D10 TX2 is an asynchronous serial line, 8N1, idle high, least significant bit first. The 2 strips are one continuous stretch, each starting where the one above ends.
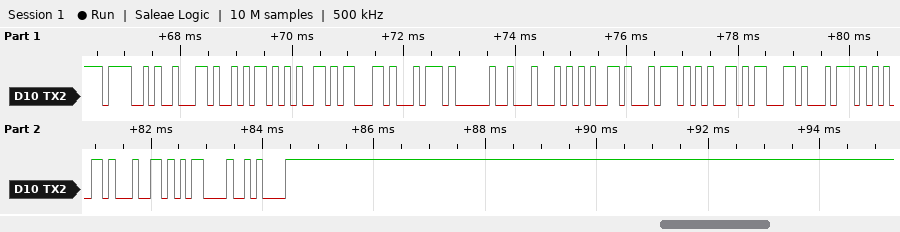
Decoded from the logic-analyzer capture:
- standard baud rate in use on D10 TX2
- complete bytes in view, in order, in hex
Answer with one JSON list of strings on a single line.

["9600 baud", "0x4F 0x62 0x6A 0x65 0x63 0x74 0x20 0x44 0x65 0x74 0x65 0x63 0x74 0x65 0x64 0x0D 0x0A"]
